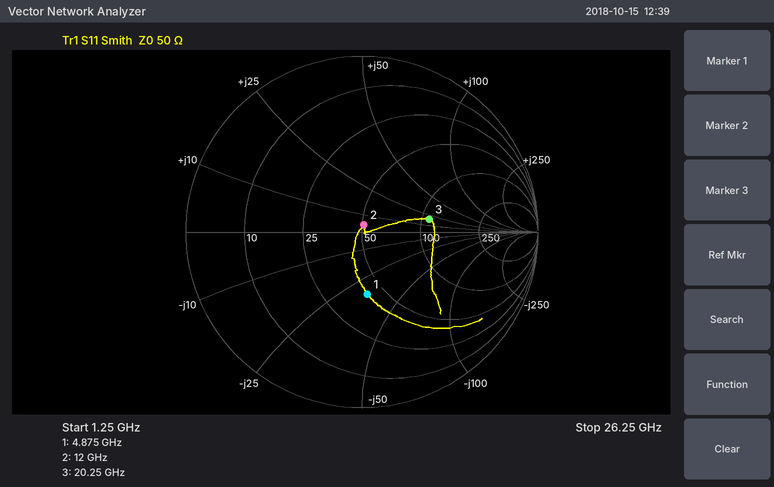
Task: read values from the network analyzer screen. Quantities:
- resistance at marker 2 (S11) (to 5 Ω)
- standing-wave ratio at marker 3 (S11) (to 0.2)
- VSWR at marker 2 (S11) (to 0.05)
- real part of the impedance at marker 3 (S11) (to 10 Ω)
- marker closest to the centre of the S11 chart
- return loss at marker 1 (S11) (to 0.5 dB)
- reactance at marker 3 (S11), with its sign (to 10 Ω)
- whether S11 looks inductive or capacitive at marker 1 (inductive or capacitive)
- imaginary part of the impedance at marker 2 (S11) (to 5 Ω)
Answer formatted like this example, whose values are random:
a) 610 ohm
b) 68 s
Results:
a) 50 Ω
b) 2.2
c) 1.10
d) 110 Ω
e) marker 2
f) 9.0 dB
g) +20 Ω
h) capacitive
i) +5 Ω
